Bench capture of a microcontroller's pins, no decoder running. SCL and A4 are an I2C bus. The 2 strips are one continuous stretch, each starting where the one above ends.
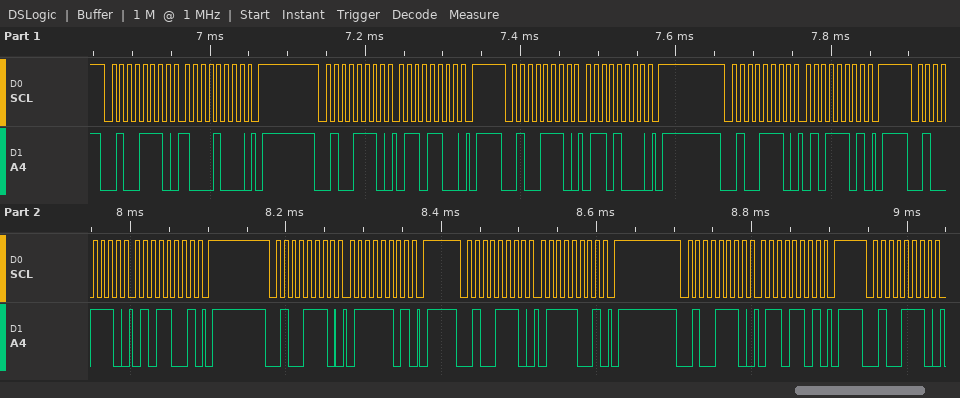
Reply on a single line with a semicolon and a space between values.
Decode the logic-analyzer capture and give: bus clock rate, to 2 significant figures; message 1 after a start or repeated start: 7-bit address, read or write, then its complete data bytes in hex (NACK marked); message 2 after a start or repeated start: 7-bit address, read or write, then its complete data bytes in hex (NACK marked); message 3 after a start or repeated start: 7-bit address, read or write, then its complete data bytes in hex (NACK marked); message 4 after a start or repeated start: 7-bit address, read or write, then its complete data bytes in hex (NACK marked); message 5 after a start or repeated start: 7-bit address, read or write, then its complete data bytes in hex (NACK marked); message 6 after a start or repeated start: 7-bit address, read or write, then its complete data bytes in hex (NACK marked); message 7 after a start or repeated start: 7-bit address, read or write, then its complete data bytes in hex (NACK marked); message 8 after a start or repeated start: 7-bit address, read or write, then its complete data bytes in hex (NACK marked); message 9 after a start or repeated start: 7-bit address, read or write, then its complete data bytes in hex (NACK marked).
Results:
100 kHz; 0x27 write: 88; 0x27 write: 6C; 0x27 write: 68; 0x27 write: 5D; 0x27 write: 59; 0x27 write: 7D; 0x27 write: 79; 0x27 write: 6D; 0x27 write
